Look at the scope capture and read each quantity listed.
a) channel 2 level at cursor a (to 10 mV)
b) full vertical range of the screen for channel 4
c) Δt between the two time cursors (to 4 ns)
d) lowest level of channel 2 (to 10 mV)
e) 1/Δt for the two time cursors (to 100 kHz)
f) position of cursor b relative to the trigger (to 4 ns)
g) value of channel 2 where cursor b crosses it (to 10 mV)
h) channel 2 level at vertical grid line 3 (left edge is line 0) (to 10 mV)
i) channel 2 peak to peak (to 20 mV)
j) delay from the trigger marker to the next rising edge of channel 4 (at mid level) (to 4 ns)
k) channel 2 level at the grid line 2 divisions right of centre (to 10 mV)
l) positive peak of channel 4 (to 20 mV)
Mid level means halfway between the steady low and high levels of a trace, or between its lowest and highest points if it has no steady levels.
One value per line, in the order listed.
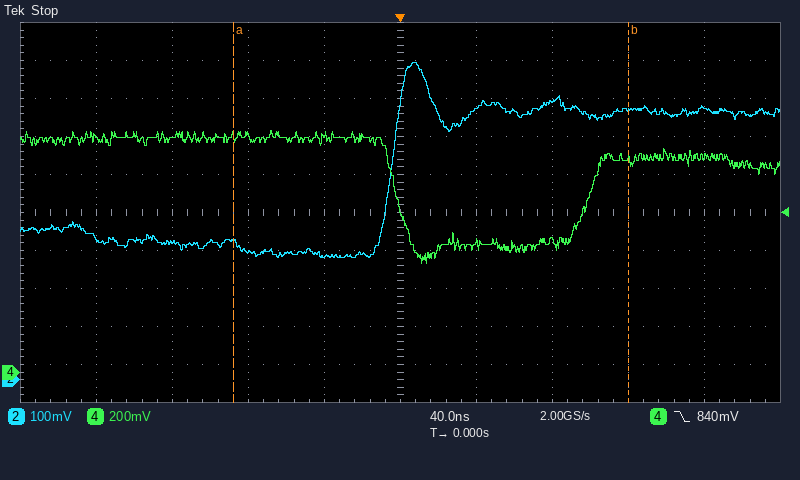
360 mV
2 V
208 ns
320 mV
4.8 MHz
+120 ns
710 mV
340 mV
520 mV
100 ns
730 mV
1.28 V
